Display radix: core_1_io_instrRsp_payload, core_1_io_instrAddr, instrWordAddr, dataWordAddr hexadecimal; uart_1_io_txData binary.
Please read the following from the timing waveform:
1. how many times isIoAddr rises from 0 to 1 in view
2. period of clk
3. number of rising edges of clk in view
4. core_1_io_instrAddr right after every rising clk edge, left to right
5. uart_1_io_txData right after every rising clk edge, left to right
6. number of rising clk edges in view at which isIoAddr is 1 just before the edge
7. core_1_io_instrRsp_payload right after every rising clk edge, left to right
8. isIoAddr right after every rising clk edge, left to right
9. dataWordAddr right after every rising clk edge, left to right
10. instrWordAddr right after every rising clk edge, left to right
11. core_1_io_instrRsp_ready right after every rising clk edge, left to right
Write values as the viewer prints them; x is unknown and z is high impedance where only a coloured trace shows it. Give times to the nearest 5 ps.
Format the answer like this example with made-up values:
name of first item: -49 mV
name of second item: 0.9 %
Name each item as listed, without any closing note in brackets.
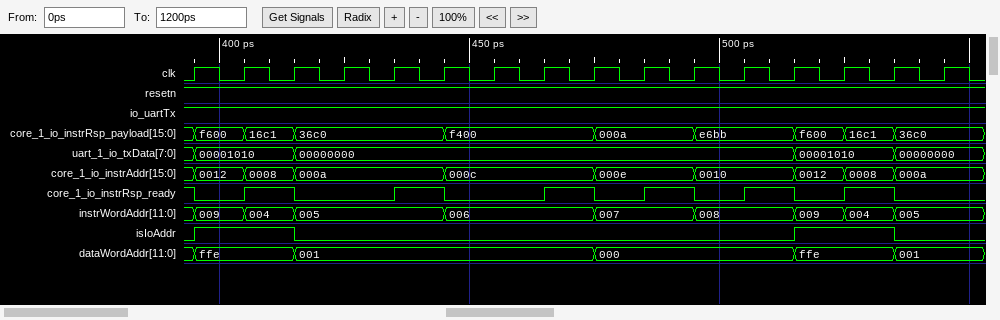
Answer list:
how many times isIoAddr rises from 0 to 1 in view: 2
period of clk: 10 ps
number of rising edges of clk in view: 16
core_1_io_instrAddr right after every rising clk edge, left to right: 0012, 0008, 000a, 000a, 000a, 000c, 000c, 000c, 000e, 000e, 0010, 0010, 0012, 0008, 000a, 000a
uart_1_io_txData right after every rising clk edge, left to right: 00001010, 00001010, 00000000, 00000000, 00000000, 00000000, 00000000, 00000000, 00000000, 00000000, 00000000, 00000000, 00001010, 00001010, 00000000, 00000000
number of rising clk edges in view at which isIoAddr is 1 just before the edge: 4
core_1_io_instrRsp_payload right after every rising clk edge, left to right: f600, 16c1, 36c0, 36c0, 36c0, f400, f400, f400, 000a, 000a, e6bb, e6bb, f600, 16c1, 36c0, 36c0
isIoAddr right after every rising clk edge, left to right: 1 1 0 0 0 0 0 0 0 0 0 0 1 1 0 0
dataWordAddr right after every rising clk edge, left to right: ffe, ffe, 001, 001, 001, 001, 001, 001, 000, 000, 000, 000, ffe, ffe, 001, 001
instrWordAddr right after every rising clk edge, left to right: 009, 004, 005, 005, 005, 006, 006, 006, 007, 007, 008, 008, 009, 004, 005, 005
core_1_io_instrRsp_ready right after every rising clk edge, left to right: 0 1 0 0 1 0 0 1 0 1 0 1 0 1 0 0
